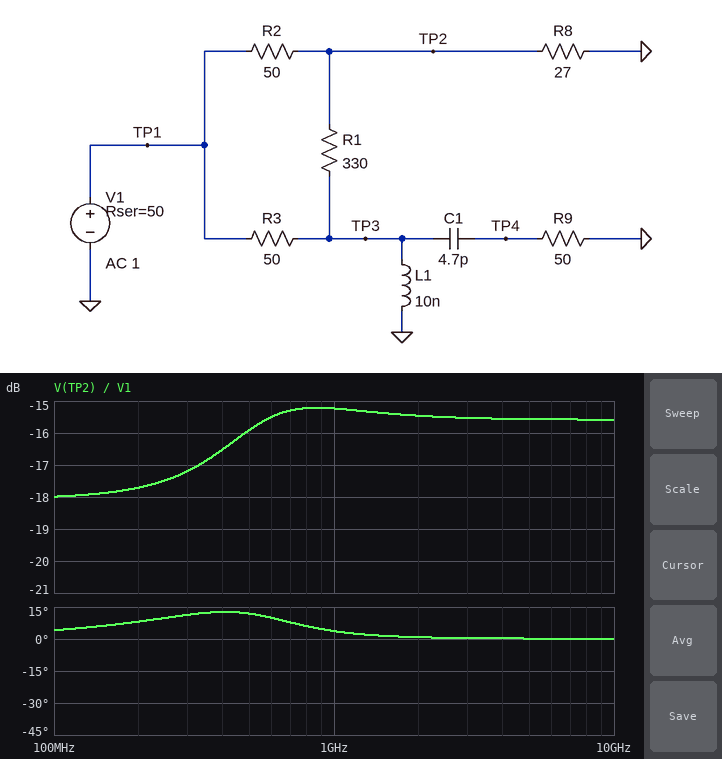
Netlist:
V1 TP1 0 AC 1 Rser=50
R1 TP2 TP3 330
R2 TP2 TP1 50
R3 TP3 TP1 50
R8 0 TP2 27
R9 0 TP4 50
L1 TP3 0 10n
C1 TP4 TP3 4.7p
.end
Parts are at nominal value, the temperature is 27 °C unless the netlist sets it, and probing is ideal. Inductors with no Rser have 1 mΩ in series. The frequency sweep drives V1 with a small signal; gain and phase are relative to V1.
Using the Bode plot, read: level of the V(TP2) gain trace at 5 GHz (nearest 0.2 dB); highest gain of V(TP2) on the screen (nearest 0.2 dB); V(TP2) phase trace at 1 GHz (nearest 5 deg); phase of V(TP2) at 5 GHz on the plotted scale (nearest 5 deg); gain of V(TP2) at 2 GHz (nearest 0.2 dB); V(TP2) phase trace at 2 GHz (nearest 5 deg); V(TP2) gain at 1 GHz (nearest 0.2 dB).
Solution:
-15.6 dB
-15.2 dB
5 deg
0 deg
-15.4 dB
0 deg
-15.2 dB
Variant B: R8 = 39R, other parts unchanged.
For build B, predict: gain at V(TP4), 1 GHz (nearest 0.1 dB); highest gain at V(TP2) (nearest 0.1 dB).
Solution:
-12.5 dB
-13.0 dB
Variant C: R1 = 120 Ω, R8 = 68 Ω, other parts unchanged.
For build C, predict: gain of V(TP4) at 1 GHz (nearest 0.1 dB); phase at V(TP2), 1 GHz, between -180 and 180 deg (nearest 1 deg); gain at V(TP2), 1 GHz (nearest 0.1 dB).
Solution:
-11.7 dB
5 deg
-10.1 dB
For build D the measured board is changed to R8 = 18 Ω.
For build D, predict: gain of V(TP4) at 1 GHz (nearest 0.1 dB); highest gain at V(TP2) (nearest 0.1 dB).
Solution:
-13.5 dB
-17.9 dB
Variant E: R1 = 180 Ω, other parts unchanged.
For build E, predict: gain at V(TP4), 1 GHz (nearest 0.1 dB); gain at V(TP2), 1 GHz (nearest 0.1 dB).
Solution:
-13.2 dB
-15.1 dB
